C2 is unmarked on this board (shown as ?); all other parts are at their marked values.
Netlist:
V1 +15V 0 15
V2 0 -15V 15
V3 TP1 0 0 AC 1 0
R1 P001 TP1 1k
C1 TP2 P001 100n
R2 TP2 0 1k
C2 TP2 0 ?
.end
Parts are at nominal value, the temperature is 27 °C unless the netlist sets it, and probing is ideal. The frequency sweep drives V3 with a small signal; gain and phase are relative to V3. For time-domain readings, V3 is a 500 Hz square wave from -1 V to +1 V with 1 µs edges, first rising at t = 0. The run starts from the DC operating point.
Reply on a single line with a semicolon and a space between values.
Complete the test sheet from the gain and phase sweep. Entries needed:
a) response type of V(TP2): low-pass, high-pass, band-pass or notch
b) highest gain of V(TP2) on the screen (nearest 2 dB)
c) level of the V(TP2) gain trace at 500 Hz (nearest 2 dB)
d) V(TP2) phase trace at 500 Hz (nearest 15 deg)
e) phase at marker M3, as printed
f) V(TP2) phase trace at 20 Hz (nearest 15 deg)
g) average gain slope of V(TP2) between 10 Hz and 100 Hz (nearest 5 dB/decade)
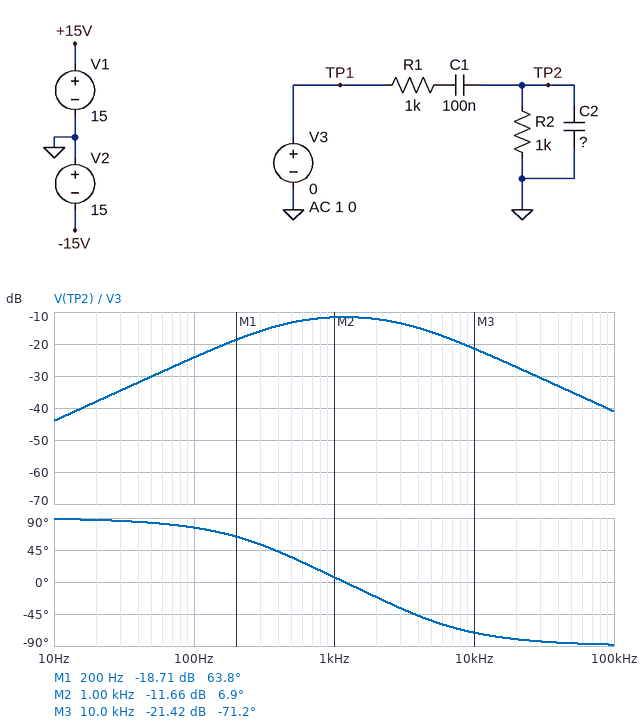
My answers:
band-pass; -12 dB; -14 dB; 30 deg; -71.2 deg; 90 deg; 20 dB/decade
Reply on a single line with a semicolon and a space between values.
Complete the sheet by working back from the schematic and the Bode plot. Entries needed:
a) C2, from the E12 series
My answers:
180 nF
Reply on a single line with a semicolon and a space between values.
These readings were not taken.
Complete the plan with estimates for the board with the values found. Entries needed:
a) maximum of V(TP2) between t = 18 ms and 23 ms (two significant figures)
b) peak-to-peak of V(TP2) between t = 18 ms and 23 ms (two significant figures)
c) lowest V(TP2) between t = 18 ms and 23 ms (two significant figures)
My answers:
410 mV; 810 mV; -410 mV
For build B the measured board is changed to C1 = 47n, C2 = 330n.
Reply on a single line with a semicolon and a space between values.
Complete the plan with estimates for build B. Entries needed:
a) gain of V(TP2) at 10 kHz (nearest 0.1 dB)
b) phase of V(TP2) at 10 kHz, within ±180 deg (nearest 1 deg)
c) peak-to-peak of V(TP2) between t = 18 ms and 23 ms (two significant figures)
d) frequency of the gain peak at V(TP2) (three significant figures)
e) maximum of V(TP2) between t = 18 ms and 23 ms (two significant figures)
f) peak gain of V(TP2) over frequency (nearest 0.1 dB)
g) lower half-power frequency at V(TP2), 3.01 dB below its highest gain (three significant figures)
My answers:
-27.0 dB; -66 deg; 350 mV; 1.28 kHz; 170 mV; -19.1 dB; 348 Hz
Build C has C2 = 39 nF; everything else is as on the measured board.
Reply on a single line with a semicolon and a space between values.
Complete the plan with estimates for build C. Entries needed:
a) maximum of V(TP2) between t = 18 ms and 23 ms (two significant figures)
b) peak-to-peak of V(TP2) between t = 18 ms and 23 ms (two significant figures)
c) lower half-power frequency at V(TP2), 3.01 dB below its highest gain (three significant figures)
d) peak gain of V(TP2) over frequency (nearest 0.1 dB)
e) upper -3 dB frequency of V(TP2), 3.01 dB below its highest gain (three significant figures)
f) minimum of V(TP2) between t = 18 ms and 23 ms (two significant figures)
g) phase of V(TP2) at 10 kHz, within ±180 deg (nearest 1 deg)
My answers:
720 mV; 1.4 V; 626 Hz; -7.6 dB; 10.4 kHz; -720 mV; -44 deg
